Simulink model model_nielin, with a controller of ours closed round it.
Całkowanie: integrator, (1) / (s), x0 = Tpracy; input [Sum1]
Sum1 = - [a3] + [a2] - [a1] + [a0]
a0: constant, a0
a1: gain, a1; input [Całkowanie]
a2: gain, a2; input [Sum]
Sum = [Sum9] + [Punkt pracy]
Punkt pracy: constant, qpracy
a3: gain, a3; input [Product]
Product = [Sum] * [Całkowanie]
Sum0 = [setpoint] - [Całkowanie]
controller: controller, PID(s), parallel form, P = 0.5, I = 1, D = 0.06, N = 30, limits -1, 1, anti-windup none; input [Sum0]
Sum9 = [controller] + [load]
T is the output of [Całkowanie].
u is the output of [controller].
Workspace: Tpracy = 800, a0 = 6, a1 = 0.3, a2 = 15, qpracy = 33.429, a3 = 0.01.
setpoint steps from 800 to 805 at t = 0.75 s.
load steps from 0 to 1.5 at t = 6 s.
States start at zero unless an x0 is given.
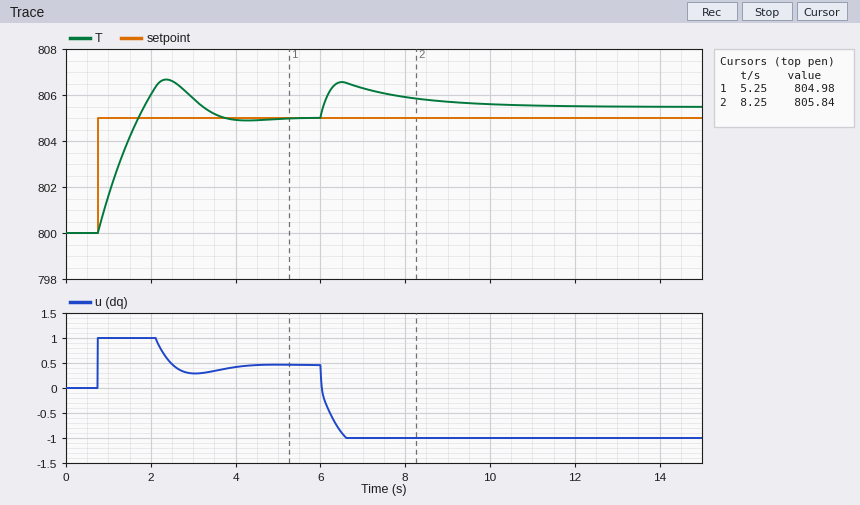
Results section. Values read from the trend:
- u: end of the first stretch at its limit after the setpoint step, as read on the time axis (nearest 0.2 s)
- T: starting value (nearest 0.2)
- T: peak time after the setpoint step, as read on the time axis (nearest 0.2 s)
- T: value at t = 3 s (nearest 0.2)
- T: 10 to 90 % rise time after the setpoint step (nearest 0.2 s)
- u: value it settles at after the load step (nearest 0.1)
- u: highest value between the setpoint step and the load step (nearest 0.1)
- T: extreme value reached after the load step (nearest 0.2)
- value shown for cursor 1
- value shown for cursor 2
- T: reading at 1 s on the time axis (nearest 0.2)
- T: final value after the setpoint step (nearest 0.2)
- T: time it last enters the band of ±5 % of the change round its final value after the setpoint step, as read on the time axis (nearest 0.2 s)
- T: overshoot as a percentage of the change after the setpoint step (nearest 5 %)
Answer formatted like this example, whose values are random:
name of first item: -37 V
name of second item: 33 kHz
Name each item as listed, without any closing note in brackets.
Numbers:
u: end of the first stretch at its limit after the setpoint step, as read on the time axis: 2.2 s
T: starting value: 800.0
T: peak time after the setpoint step, as read on the time axis: 2.4 s
T: value at t = 3 s: 805.8
T: 10 to 90 % rise time after the setpoint step: 0.8 s
u: value it settles at after the load step: -1.0
u: highest value between the setpoint step and the load step: 1.0
T: extreme value reached after the load step: 806.6
value shown for cursor 1: 804.98
value shown for cursor 2: 805.84
T: reading at 1 s on the time axis: 801.6
T: final value after the setpoint step: 805.0
T: time it last enters the band of ±5 % of the change round its final value after the setpoint step, as read on the time axis: 3.4 s
T: overshoot as a percentage of the change after the setpoint step: 35 %
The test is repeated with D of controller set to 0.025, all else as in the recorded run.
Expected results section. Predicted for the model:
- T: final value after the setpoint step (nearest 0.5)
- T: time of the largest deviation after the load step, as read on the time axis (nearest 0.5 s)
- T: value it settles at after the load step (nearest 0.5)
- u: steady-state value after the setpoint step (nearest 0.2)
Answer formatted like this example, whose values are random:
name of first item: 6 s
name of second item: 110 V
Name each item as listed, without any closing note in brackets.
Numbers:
T: final value after the setpoint step: 805.0
T: time of the largest deviation after the load step, as read on the time axis: 6.5 s
T: value it settles at after the load step: 805.5
u: steady-state value after the setpoint step: 0.4
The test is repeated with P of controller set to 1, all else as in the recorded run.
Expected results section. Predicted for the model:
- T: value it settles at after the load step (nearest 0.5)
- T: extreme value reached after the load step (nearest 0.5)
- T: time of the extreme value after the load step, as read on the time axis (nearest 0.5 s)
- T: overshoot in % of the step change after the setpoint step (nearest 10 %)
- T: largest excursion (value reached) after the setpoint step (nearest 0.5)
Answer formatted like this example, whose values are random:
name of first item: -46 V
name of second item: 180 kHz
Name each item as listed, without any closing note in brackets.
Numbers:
T: value it settles at after the load step: 805.5
T: extreme value reached after the load step: 806.0
T: time of the extreme value after the load step, as read on the time axis: 6.5 s
T: overshoot in % of the step change after the setpoint step: 20 %
T: largest excursion (value reached) after the setpoint step: 806.0
